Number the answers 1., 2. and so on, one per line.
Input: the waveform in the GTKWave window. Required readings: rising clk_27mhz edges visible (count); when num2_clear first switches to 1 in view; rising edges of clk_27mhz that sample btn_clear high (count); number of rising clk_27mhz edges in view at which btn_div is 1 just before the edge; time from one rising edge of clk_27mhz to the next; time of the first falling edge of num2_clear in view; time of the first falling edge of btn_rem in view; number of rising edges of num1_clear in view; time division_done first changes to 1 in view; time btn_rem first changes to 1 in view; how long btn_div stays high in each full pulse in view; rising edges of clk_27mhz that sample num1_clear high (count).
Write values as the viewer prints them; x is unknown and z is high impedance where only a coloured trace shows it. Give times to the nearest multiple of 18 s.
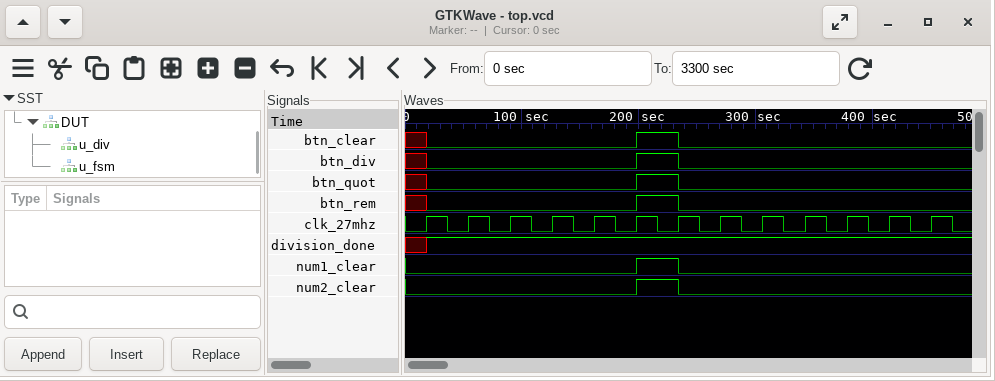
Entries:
1. 13
2. 198 s
3. 1
4. 1
5. 36 s
6. 234 s
7. 234 s
8. 1
9. 18 s
10. 198 s
11. 36 s
12. 1
